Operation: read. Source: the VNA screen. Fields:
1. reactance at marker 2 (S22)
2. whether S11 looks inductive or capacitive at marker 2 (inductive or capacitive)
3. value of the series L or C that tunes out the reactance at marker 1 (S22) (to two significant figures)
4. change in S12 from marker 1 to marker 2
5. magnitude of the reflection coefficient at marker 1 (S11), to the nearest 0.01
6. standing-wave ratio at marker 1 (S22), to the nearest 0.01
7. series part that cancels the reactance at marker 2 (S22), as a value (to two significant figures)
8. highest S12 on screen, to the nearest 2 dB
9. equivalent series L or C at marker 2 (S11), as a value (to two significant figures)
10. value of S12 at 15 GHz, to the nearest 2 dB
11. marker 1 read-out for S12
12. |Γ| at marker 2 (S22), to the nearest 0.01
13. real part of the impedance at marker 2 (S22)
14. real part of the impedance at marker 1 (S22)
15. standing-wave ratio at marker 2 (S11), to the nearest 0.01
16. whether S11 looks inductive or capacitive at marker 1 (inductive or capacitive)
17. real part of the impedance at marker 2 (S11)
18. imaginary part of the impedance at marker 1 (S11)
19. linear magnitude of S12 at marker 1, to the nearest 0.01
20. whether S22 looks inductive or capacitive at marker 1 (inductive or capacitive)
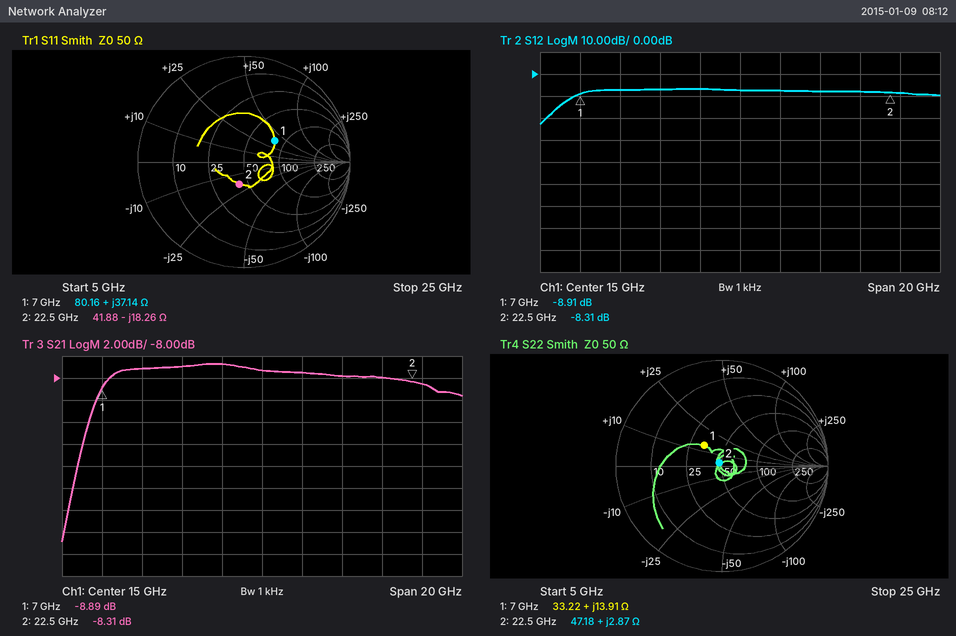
+2.87 Ω
capacitive
1.6 pF
0.60 dB
0.35
1.70
2.5 pF
-6 dB
390 fF
-8 dB
-8.91 dB
0.04
47.18 Ω
33.22 Ω
1.54
inductive
41.88 Ω
+37.14 Ω
0.36
inductive
